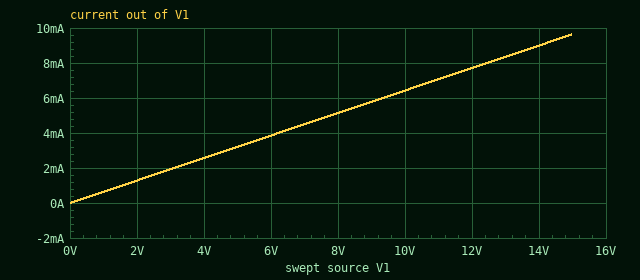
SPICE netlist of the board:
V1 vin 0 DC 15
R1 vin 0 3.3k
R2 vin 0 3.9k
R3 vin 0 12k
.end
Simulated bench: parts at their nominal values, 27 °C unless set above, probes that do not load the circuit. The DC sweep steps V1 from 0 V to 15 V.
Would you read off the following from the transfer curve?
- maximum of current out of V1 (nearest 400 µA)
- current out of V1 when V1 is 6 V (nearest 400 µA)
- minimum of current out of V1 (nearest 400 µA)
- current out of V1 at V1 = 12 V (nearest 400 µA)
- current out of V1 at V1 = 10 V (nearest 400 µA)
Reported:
9.6 mA
4.0 mA
0 A
7.6 mA
6.4 mA
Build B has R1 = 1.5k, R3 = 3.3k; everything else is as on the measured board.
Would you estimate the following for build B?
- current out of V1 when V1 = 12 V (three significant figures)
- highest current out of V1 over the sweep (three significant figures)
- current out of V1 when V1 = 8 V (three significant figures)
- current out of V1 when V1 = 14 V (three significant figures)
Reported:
14.7 mA
18.4 mA
9.81 mA
17.2 mA
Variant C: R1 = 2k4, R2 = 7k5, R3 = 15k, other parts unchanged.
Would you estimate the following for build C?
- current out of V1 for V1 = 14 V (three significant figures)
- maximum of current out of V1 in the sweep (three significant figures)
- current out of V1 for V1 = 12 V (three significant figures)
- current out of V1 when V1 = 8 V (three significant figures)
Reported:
8.63 mA
9.25 mA
7.40 mA
4.93 mA
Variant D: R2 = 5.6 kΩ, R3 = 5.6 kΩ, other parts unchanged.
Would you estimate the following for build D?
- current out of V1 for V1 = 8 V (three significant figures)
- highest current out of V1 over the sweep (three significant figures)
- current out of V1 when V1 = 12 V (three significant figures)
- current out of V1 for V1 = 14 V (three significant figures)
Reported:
5.28 mA
9.90 mA
7.92 mA
9.24 mA
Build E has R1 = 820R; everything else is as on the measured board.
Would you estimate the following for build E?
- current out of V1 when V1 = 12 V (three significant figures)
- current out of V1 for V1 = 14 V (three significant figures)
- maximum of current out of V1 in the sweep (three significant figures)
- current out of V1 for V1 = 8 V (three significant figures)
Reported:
18.7 mA
21.8 mA
23.4 mA
12.5 mA
